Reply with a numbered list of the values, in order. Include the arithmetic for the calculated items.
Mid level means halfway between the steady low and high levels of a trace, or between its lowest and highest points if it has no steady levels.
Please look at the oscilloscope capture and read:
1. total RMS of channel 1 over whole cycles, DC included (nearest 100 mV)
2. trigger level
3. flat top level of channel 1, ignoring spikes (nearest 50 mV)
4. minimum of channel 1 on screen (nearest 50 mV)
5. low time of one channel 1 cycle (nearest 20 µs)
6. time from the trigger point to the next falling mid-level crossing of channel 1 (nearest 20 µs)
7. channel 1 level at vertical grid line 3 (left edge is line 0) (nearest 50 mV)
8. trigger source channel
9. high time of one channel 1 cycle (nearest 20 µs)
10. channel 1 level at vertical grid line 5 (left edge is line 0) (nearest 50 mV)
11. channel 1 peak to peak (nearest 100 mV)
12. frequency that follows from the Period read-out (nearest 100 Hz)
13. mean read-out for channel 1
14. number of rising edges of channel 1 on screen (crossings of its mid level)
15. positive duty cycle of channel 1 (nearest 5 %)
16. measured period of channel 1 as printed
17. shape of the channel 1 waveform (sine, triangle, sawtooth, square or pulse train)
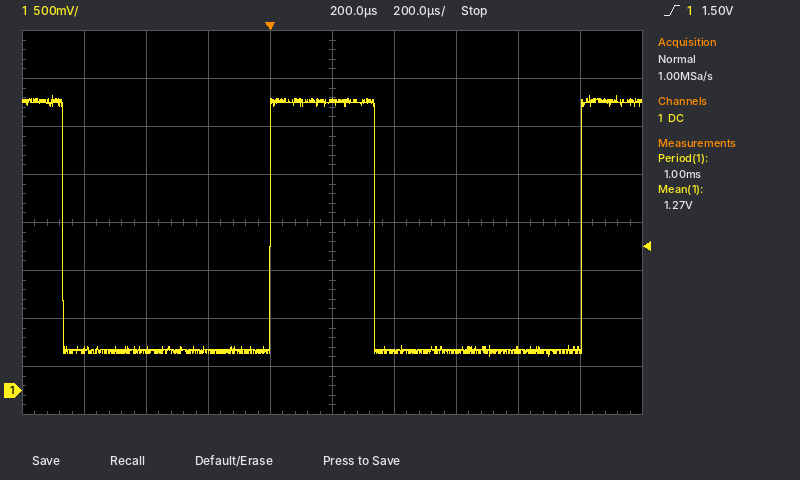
1. √(0.35 × (3.00 V)² + 0.65 × (350 mV)²) ≈ 1.8 V
2. 1.50 V
3. 3.00 V
4. 350 mV
5. 660 µs
6. 340 µs
7. 400 mV
8. channel 1
9. 340 µs
10. 3.00 V
11. 2.70 V
12. 1 / 1.00 ms ≈ 1.0 kHz
13. 1.27 V
14. 2
15. 35 %
16. 1.00 ms
17. pulse train
